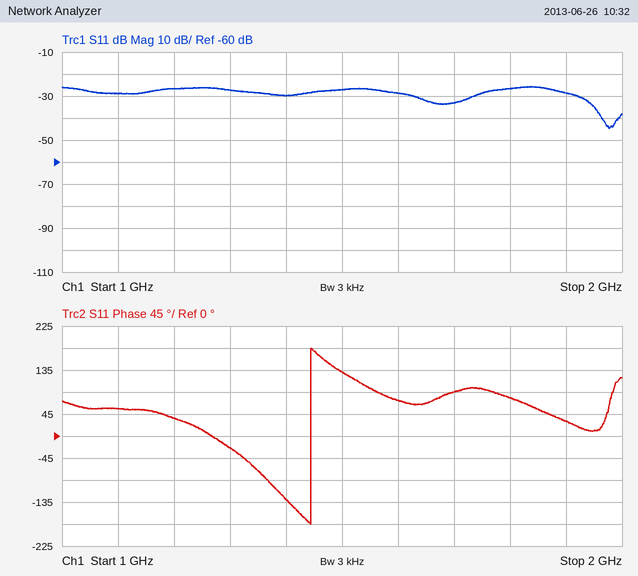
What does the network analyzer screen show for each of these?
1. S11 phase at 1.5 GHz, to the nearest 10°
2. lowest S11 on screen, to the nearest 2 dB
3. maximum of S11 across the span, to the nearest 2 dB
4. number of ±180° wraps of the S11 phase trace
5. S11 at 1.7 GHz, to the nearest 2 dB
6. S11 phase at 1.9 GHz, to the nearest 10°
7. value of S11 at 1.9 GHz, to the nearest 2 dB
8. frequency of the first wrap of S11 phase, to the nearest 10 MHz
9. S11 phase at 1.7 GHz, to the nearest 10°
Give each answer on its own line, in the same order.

130°
-44 dB
-26 dB
1
-34 dB
30°
-28 dB
1.44 GHz
90°
